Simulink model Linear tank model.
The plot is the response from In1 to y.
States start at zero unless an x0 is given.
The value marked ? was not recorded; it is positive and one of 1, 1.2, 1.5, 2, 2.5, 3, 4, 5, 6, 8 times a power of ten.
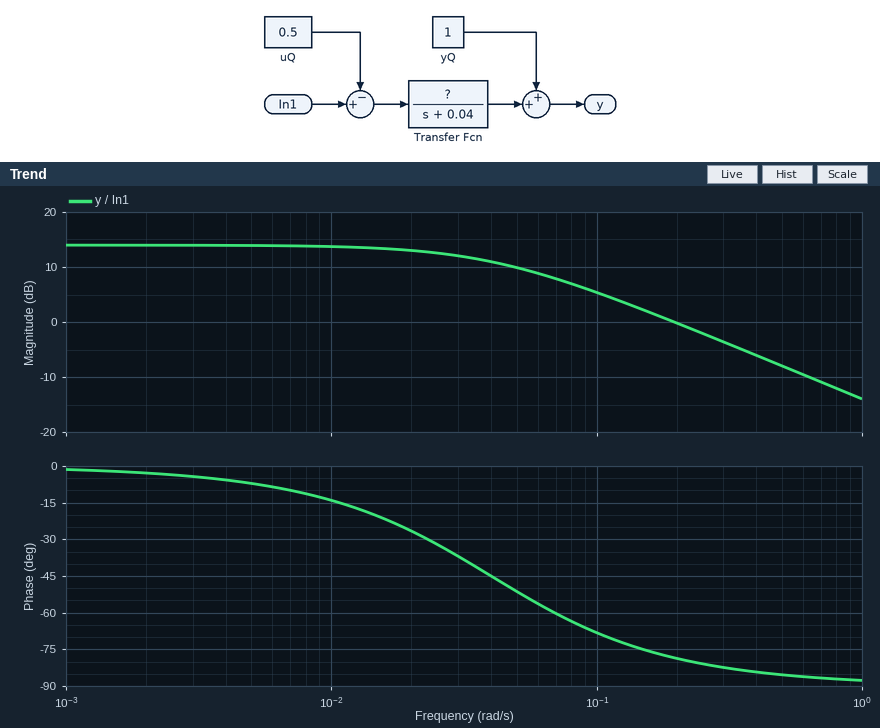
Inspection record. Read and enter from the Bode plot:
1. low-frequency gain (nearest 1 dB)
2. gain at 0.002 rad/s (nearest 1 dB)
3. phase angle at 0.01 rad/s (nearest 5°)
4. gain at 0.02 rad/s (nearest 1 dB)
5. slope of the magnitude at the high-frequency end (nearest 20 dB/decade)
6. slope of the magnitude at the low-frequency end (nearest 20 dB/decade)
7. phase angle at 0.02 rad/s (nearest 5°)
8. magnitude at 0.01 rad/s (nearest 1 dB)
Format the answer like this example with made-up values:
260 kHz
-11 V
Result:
14 dB
14 dB
-15°
13 dB
-20 dB/decade
0 dB/decade
-25°
14 dB
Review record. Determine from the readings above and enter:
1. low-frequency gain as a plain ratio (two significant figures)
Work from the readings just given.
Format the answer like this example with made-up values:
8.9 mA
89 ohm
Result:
5.0
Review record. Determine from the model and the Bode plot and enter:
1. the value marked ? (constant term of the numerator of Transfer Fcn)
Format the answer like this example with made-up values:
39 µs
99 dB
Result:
0.2
